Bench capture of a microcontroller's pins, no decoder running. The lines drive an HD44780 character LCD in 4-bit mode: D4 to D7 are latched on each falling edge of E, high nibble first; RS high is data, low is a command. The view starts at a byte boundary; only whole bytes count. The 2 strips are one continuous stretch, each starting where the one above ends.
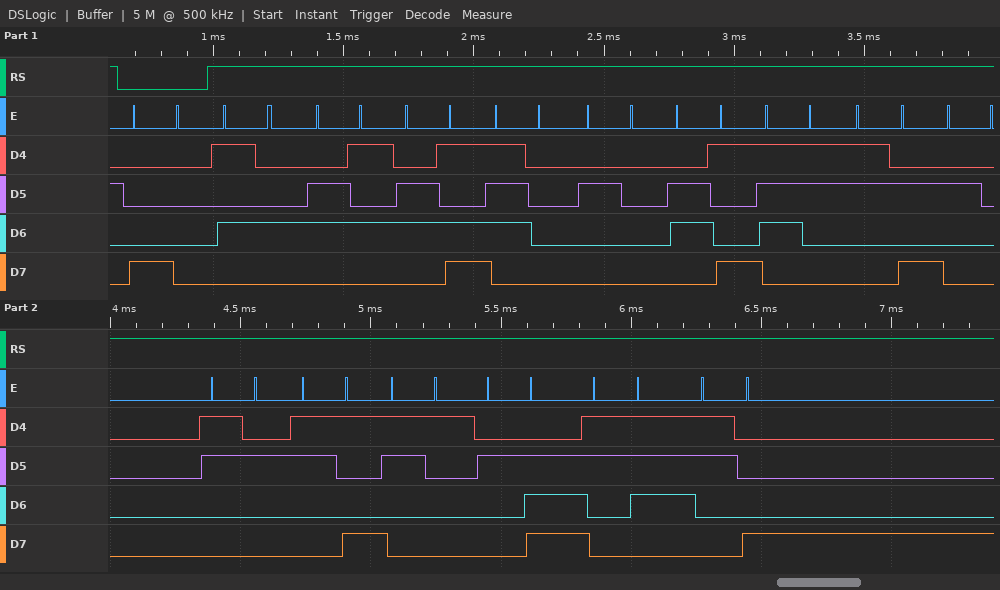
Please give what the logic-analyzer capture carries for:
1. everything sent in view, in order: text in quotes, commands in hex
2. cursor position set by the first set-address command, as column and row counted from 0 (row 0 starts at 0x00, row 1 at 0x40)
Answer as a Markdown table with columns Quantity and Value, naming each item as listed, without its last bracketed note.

| Quantity | Value |
|---|---|
| everything sent in view, in order: text in quotes, commands in hex | 0x80 "Temp is: 291.78" |
| cursor position set by the first set-address command, as column and row counted from 0 | column 0, row 0 |
